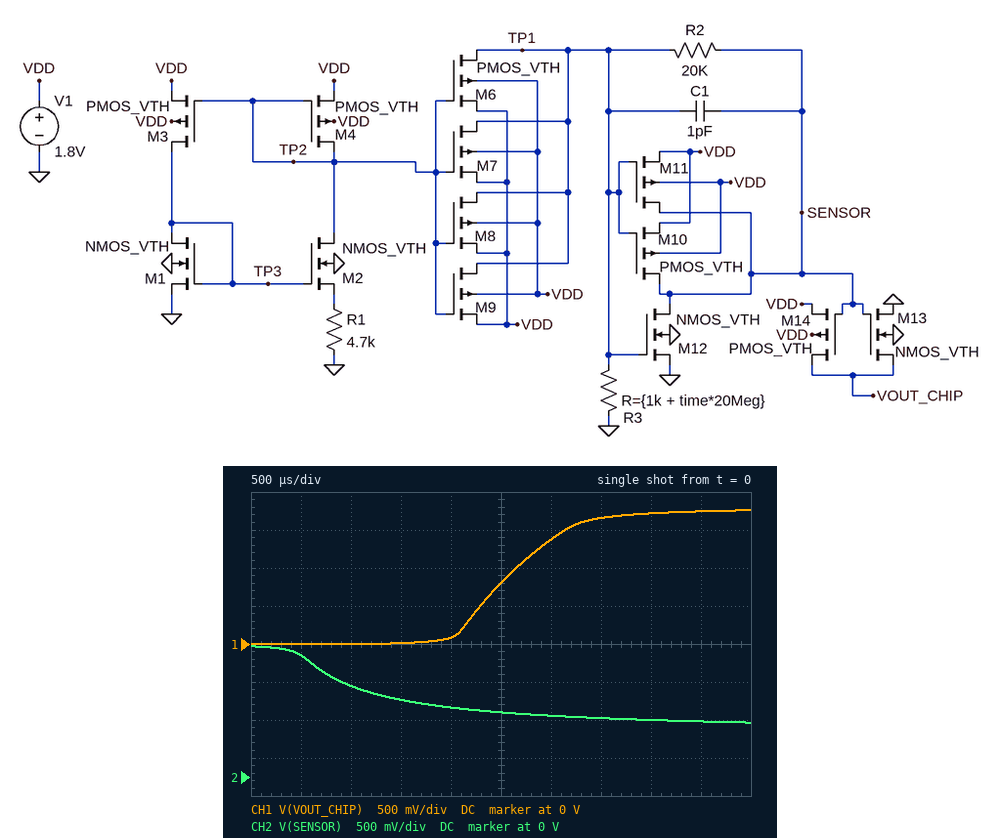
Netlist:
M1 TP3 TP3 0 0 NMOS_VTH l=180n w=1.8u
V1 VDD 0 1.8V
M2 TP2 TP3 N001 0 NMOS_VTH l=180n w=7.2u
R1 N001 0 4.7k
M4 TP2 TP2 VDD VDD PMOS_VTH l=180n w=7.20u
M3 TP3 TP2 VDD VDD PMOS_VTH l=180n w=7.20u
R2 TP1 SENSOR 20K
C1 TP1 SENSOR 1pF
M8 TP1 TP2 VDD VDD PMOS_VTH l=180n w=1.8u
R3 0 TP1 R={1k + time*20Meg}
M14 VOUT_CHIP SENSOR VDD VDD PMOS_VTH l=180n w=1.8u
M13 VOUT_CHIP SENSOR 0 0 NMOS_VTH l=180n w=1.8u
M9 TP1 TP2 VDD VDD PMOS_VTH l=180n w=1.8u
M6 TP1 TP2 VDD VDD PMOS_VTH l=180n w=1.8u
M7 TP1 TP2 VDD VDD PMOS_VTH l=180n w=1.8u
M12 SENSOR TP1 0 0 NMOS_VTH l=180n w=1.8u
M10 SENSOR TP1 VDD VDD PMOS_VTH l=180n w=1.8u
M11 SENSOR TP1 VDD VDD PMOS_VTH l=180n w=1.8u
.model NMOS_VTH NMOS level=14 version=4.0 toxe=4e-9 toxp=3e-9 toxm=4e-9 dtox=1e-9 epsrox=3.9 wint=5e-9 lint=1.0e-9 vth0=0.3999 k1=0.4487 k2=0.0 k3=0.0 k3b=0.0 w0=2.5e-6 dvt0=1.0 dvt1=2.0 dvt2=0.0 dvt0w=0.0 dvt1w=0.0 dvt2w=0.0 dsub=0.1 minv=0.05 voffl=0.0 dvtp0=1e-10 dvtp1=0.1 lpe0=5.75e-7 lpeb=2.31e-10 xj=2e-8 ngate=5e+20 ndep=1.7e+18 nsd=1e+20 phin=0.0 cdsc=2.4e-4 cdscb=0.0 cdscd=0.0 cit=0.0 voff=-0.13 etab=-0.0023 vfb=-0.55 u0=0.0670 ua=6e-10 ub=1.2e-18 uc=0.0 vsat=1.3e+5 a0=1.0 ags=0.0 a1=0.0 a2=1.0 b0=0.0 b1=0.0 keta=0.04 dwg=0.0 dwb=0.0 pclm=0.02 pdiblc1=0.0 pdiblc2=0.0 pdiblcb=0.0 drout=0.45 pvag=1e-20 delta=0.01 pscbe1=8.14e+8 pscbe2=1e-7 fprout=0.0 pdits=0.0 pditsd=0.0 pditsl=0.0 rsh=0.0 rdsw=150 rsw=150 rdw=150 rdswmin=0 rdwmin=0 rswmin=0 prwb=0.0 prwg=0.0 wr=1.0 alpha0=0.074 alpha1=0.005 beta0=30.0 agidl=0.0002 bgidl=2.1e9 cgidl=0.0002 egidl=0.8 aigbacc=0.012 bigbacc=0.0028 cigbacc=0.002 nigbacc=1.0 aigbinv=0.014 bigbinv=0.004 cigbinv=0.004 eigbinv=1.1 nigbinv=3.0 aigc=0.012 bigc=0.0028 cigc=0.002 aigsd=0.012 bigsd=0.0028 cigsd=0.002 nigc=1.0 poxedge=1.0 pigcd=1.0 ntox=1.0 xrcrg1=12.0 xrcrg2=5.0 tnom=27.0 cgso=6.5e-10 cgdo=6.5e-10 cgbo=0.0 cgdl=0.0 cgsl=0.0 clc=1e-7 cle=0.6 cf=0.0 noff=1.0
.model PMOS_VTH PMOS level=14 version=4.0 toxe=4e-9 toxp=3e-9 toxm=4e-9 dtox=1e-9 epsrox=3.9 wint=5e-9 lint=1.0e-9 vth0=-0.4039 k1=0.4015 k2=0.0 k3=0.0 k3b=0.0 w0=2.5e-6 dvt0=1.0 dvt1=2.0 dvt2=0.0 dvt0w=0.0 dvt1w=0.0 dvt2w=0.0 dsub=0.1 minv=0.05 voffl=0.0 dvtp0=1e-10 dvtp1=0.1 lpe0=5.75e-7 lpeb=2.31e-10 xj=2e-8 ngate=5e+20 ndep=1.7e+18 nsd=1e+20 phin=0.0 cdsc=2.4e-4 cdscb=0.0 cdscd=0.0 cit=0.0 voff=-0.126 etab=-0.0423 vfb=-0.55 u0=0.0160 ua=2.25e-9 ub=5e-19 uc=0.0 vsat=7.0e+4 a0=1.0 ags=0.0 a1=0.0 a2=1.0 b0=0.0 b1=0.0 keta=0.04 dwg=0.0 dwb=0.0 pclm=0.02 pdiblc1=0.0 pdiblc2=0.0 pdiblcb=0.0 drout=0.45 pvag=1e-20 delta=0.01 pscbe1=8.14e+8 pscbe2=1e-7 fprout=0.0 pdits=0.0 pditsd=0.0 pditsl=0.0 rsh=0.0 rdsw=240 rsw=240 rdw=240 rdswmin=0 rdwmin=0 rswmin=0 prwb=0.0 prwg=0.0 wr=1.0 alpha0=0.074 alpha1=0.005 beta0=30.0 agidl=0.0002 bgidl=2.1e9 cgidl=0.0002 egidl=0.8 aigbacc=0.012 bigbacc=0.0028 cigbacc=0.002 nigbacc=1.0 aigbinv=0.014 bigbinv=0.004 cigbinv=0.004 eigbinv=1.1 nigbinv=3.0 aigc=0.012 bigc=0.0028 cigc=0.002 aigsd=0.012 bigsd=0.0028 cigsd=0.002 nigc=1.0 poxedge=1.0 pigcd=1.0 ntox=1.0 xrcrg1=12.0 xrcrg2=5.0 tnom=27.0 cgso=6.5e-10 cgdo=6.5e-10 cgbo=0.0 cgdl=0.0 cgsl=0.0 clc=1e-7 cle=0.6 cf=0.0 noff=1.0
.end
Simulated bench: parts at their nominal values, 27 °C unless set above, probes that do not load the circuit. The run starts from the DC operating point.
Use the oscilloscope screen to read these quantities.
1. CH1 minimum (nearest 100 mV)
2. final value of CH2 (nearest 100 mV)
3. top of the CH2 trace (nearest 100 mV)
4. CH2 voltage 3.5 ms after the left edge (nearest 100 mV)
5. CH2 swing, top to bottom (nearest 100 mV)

0 V
700 mV
1.7 V
800 mV
1.0 V
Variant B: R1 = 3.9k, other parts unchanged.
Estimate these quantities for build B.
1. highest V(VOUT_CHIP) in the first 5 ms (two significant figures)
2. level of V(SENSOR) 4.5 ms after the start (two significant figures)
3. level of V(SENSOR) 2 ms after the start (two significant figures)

1.8 V
680 mV
860 mV
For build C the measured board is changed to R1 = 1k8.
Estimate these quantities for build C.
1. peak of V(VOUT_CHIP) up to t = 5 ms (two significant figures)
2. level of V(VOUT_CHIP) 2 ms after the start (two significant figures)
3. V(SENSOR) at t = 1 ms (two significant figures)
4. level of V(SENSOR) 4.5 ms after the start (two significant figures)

1.8 V
1.8 V
810 mV
320 mV
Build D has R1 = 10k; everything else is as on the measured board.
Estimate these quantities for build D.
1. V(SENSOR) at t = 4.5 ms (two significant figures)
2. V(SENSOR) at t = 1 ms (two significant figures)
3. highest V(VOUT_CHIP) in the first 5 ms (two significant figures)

870 mV
1.3 V
700 mV
